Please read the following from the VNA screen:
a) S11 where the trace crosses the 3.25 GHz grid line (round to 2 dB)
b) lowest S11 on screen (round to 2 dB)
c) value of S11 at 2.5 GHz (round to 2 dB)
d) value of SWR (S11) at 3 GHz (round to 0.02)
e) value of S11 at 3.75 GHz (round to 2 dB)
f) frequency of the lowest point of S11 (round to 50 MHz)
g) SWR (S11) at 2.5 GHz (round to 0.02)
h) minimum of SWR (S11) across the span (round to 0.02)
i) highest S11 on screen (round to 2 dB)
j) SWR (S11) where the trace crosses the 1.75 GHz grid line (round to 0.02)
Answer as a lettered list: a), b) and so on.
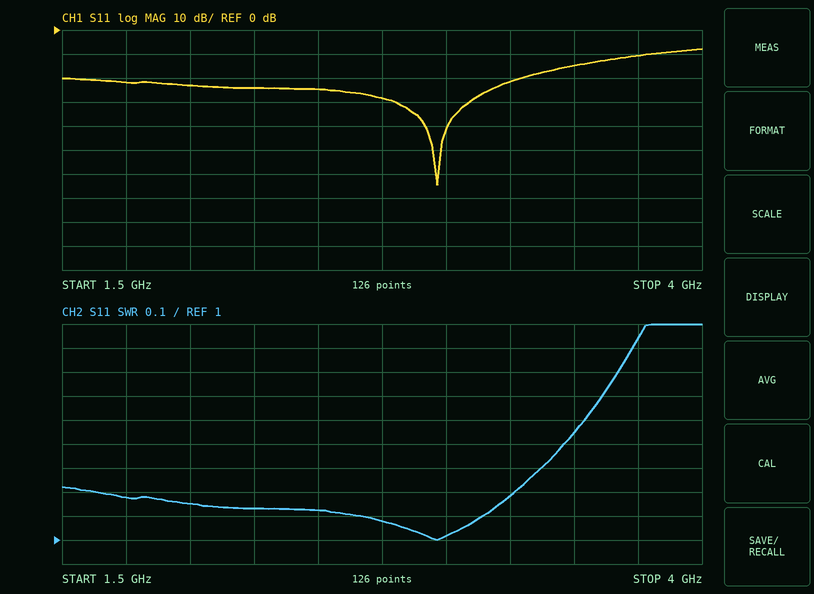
a) -22 dB
b) -64 dB
c) -24 dB
d) 1.02
e) -10 dB
f) 2.95 GHz
g) 1.12
h) 1.00
i) -8 dB
j) 1.18
